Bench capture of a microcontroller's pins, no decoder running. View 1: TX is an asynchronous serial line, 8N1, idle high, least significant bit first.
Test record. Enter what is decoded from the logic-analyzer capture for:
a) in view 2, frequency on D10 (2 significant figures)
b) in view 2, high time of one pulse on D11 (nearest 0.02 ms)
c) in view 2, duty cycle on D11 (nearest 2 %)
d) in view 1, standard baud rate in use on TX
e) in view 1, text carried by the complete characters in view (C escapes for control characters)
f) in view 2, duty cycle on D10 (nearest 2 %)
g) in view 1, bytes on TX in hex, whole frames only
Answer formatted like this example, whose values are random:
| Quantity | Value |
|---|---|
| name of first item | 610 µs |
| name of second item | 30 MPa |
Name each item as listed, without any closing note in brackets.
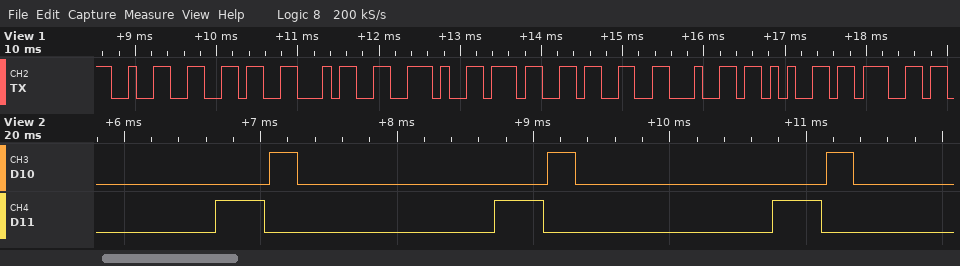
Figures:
| Quantity | Value |
|---|---|
| in view 2, frequency on D10 | 490 Hz |
| in view 2, high time of one pulse on D11 | 0.36 ms |
| in view 2, duty cycle on D11 | 18 % |
| in view 1, standard baud rate in use on TX | 9600 baud |
| in view 1, text carried by the complete characters in view | "264.73deg" |
| in view 2, duty cycle on D10 | 10 % |
| in view 1, bytes on TX in hex, whole frames only | 32 36 34 2E 37 33 64 65 67 |
